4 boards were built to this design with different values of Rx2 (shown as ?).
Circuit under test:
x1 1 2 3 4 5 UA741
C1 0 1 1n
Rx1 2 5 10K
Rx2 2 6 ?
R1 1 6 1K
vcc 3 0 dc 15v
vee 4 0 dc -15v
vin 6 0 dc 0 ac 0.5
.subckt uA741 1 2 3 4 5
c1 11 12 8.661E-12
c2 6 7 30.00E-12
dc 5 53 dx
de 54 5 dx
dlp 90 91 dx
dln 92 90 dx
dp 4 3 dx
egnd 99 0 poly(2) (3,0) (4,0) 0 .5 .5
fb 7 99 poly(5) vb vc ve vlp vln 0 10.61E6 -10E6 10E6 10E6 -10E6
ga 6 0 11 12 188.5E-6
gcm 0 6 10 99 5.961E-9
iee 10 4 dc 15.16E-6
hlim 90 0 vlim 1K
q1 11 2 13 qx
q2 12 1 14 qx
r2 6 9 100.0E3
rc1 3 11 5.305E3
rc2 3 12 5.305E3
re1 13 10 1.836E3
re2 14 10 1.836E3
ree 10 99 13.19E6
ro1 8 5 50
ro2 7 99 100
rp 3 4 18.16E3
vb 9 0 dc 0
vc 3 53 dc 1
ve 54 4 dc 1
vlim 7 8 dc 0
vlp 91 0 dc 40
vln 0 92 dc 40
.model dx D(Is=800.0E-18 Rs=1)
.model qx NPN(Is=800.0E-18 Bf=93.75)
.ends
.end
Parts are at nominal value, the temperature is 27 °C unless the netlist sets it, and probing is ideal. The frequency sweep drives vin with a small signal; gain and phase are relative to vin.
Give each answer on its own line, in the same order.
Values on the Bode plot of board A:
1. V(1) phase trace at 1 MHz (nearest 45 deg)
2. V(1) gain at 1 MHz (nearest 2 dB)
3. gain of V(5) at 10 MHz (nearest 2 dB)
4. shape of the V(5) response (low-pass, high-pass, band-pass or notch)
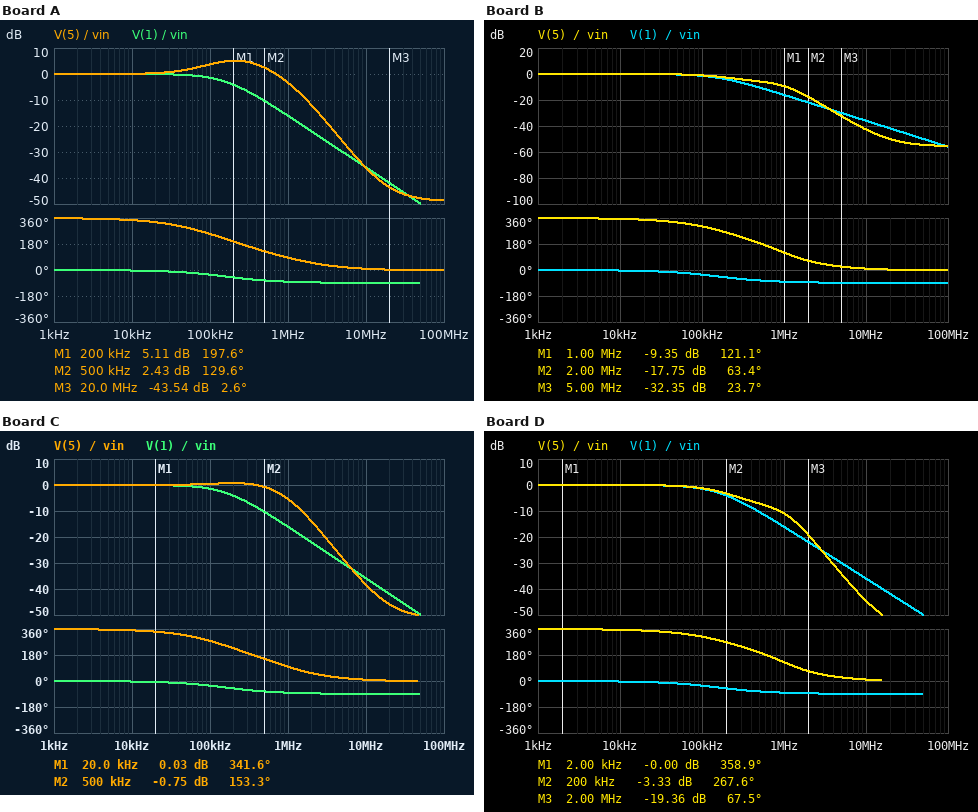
-90 deg
-16 dB
-36 dB
low-pass
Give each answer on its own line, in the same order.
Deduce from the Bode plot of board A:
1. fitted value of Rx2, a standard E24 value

3.9 kΩ
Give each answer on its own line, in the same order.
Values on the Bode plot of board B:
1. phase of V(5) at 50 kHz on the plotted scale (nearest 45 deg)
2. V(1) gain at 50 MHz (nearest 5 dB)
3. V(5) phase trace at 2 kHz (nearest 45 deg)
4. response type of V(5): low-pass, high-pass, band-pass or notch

315 deg
-50 dB
360 deg
low-pass
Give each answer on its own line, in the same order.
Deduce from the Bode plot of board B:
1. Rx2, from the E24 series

20 kΩ
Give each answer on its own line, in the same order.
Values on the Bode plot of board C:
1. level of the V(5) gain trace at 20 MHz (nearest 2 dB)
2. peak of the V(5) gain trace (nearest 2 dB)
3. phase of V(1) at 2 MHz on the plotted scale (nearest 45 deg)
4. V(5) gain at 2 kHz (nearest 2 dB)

-46 dB
0 dB
-90 deg
0 dB
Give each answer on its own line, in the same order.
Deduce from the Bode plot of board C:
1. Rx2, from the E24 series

8.2 kΩ
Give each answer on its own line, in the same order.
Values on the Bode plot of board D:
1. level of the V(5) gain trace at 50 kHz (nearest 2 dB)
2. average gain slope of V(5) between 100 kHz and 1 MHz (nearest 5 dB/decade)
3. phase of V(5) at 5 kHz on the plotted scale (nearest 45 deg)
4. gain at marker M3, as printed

0 dB
-10 dB/decade
360 deg
-19.36 dB
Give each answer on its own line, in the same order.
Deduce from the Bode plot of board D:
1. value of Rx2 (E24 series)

27 kΩ
